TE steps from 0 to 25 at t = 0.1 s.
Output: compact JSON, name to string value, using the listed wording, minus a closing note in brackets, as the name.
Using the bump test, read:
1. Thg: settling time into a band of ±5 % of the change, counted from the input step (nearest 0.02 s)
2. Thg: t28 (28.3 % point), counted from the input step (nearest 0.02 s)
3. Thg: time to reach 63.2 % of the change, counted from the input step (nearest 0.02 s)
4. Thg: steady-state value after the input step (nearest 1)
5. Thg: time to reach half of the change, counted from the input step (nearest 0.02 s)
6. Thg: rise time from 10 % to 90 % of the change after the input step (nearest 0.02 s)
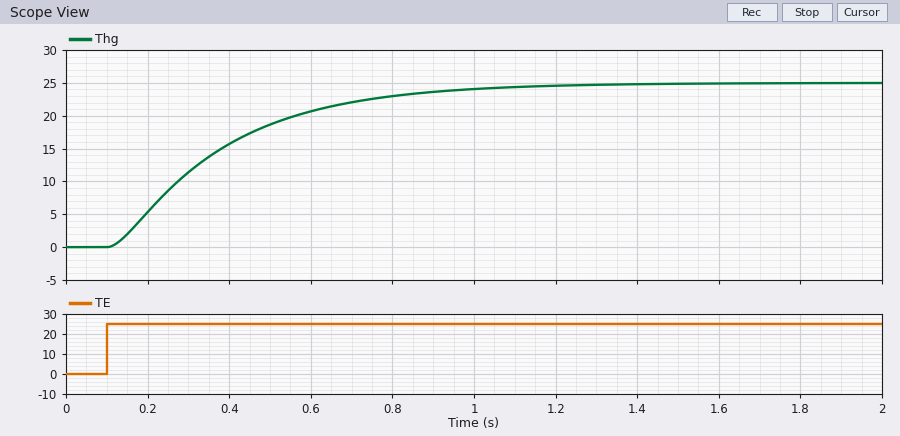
{"Thg: settling time into a band of ±5 % of the change, counted from the input step": "0.82 s", "Thg: t28 (28.3 % point), counted from the input step": "0.12 s", "Thg: time to reach 63.2 % of the change, counted from the input step": "0.30 s", "Thg: steady-state value after the input step": "25", "Thg: time to reach half of the change, counted from the input step": "0.22 s", "Thg: rise time from 10 % to 90 % of the change after the input step": "0.58 s"}
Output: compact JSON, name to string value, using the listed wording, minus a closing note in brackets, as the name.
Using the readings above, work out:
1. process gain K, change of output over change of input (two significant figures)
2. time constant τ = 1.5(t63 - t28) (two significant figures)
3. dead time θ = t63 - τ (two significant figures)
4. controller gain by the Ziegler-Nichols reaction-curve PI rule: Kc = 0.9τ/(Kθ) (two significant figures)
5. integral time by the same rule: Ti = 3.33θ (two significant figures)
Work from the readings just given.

{"process gain K, change of output over change of input": "1.0", "time constant τ = 1.5(t63 - t28)": "0.27 s", "dead time θ = t63 - τ": "0.030 s", "controller gain by the Ziegler-Nichols reaction-curve PI rule: Kc = 0.9τ/(Kθ)": "8.1", "integral time by the same rule: Ti = 3.33θ": "0.100 s"}
